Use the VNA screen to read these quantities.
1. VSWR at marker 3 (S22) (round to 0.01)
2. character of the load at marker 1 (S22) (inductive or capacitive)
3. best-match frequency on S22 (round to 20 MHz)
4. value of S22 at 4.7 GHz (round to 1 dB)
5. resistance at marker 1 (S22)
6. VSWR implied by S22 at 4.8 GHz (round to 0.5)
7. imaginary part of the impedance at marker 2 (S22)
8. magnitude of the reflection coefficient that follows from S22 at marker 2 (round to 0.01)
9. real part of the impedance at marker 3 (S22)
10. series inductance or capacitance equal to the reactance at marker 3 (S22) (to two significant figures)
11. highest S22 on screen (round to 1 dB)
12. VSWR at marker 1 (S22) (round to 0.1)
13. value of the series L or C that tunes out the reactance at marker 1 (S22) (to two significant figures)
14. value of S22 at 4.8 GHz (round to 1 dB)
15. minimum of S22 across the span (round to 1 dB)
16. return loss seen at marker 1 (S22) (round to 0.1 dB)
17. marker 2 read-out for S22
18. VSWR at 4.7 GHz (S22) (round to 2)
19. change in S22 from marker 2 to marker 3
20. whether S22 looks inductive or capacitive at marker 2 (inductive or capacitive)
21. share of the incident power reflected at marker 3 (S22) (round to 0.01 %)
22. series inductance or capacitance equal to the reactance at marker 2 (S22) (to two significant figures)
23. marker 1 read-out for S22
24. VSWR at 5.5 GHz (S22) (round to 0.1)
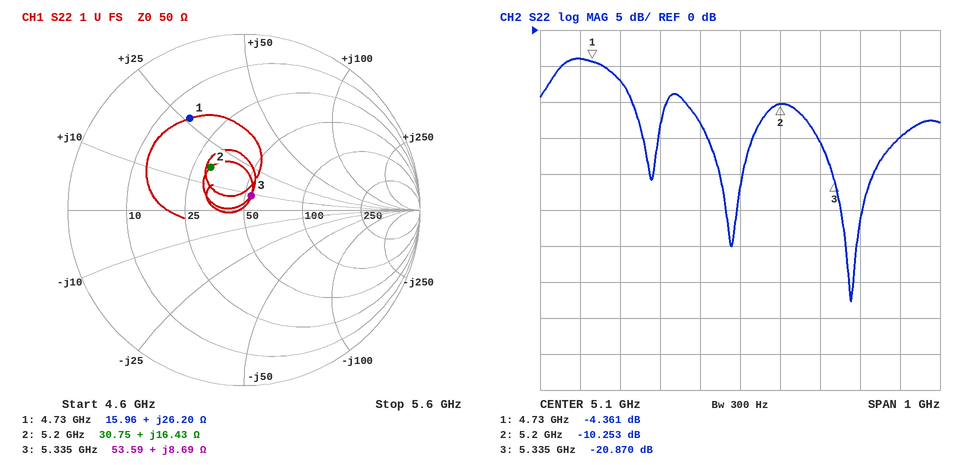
1.20
inductive
5.38 GHz
-4 dB
15.96 Ω
2.5
+16.43 Ω
0.31
53.59 Ω
260 pH
-4 dB
4.1
1.3 pF
-7 dB
-38 dB
4.4 dB
-10.253 dB
4
-10.617 dB
inductive
0.82 %
500 pH
-4.361 dB
1.4
